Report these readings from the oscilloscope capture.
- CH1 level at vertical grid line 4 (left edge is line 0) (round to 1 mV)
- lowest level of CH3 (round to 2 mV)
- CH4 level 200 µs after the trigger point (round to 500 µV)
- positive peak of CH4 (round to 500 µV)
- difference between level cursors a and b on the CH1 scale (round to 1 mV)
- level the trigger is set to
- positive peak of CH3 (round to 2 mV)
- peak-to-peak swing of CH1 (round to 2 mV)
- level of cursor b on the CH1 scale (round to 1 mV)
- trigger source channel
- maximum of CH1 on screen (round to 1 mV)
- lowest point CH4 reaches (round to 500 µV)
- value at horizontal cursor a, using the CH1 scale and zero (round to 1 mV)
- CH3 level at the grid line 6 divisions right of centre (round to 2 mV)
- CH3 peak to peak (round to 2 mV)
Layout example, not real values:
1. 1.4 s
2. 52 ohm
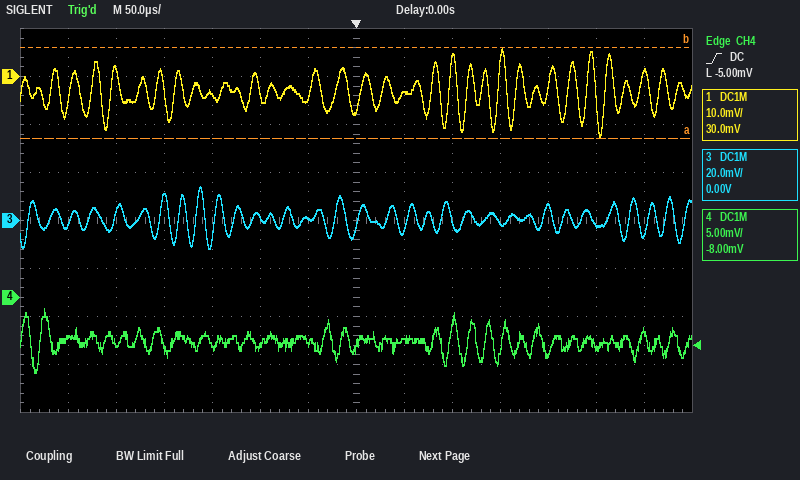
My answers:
1. -4 mV
2. -12 mV
3. -6.0 mV
4. -1.0 mV
5. 19 mV
6. -5.00 mV
7. 14 mV
8. 18 mV
9. 6 mV
10. CH4
11. 6 mV
12. -8.0 mV
13. -13 mV
14. -6 mV
15. 26 mV
